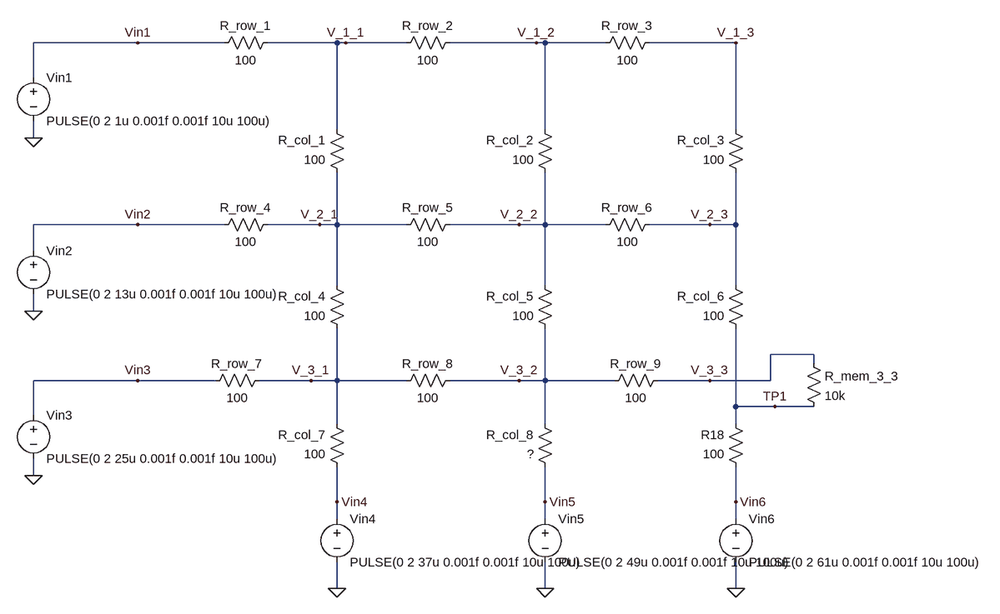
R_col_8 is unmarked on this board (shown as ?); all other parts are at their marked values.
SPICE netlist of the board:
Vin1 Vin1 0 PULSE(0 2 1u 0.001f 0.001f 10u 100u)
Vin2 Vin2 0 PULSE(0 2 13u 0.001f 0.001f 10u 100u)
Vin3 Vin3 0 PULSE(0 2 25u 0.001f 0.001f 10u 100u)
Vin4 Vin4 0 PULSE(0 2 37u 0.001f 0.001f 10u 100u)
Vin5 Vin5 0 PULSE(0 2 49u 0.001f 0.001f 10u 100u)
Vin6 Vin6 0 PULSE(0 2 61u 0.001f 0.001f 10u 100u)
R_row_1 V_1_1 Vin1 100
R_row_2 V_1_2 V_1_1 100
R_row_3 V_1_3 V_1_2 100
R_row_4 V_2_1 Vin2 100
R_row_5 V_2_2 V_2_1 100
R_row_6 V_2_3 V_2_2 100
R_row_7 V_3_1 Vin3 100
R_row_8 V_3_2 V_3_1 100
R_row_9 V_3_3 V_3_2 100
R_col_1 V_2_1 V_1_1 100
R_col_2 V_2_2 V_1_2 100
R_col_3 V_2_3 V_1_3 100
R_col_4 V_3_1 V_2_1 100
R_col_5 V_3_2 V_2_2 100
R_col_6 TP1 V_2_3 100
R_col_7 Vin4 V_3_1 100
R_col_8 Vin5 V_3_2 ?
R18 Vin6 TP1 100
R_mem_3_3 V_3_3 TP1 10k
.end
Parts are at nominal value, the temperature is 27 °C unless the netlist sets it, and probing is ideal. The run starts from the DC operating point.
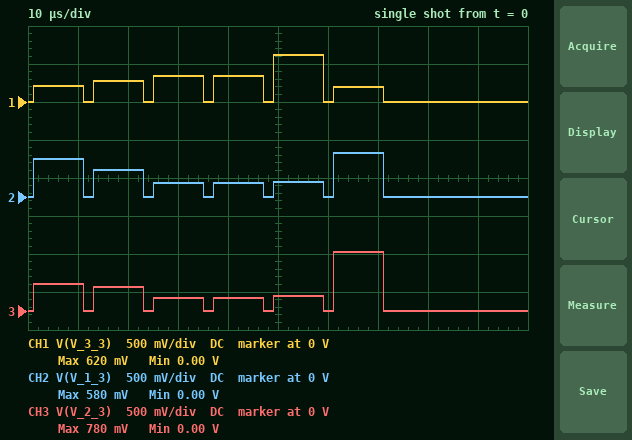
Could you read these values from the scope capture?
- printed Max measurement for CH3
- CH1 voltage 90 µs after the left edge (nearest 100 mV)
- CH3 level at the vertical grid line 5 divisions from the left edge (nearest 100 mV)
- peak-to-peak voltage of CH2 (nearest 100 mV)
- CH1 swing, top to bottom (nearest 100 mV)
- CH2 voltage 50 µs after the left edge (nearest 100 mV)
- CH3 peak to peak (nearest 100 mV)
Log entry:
780 mV
0 V
200 mV
600 mV
600 mV
200 mV
800 mV
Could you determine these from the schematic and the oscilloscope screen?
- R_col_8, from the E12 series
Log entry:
180 Ω
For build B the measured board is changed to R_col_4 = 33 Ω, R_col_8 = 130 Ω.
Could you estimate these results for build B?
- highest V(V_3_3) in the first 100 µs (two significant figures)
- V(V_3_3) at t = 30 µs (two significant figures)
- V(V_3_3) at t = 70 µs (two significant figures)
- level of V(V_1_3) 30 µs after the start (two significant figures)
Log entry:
760 mV
300 mV
180 mV
210 mV
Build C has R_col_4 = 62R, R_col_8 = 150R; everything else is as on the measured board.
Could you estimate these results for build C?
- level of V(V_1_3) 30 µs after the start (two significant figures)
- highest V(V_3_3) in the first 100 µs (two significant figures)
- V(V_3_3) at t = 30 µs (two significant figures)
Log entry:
190 mV
700 mV
320 mV
